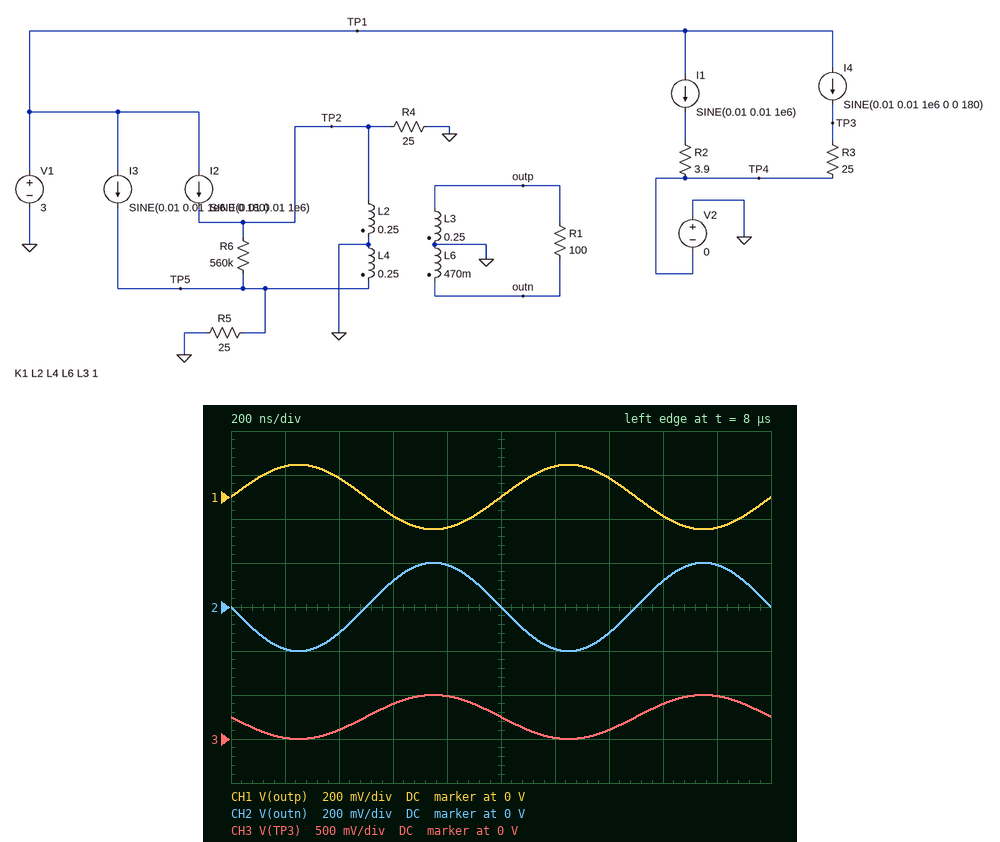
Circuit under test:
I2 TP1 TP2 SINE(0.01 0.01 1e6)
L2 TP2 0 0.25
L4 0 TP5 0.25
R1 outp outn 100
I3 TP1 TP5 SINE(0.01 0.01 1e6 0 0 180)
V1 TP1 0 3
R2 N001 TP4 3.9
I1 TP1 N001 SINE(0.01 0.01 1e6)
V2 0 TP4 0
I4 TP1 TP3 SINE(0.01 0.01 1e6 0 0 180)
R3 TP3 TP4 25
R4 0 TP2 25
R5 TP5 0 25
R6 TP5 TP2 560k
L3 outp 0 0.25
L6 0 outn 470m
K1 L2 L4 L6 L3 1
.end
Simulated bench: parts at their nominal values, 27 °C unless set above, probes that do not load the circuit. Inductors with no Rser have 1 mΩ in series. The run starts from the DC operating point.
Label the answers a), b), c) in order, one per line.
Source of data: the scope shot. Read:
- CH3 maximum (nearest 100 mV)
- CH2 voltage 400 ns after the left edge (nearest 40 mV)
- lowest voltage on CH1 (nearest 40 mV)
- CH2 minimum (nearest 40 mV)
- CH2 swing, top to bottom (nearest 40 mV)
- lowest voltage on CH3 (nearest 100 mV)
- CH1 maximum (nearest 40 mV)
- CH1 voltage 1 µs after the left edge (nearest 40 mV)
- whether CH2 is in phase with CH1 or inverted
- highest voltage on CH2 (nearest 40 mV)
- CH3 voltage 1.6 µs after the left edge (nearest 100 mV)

a) 500 mV
b) -120 mV
c) -160 mV
d) -200 mV
e) 400 mV
f) 0 V
g) 160 mV
h) 0 V
i) inverted
j) 200 mV
k) 400 mV
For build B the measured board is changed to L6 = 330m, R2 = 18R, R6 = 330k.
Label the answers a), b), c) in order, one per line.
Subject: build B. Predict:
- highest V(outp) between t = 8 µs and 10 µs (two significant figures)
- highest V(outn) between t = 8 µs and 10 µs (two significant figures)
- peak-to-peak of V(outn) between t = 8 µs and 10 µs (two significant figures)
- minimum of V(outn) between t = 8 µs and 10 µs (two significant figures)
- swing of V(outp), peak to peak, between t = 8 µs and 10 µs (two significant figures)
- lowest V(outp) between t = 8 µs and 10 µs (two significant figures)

a) 160 mV
b) 180 mV
c) 360 mV
d) -180 mV
e) 320 mV
f) -160 mV
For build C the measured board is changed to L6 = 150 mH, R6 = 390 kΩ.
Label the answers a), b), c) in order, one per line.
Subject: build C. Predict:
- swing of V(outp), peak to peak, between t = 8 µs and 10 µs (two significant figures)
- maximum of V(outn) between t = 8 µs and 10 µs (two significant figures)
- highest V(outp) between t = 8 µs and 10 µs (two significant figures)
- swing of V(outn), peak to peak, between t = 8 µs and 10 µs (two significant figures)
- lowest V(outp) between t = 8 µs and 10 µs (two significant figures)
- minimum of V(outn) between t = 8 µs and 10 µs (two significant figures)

a) 360 mV
b) 140 mV
c) 180 mV
d) 280 mV
e) -180 mV
f) -140 mV
